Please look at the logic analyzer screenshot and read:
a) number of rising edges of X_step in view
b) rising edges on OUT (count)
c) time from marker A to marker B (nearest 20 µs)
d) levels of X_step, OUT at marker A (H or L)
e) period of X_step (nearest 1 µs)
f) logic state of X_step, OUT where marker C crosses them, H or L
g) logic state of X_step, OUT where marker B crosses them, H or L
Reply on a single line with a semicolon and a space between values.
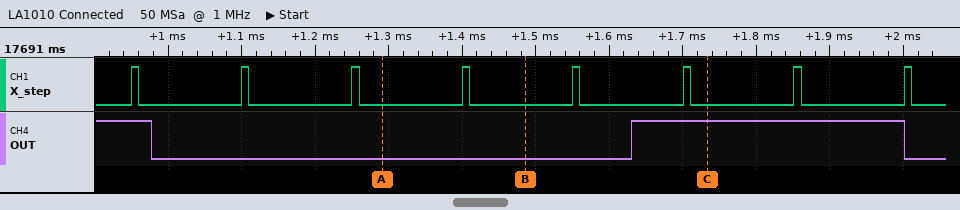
8; 1; 200 µs; X_step=L, OUT=L; 150 µs; X_step=L, OUT=H; X_step=L, OUT=L
